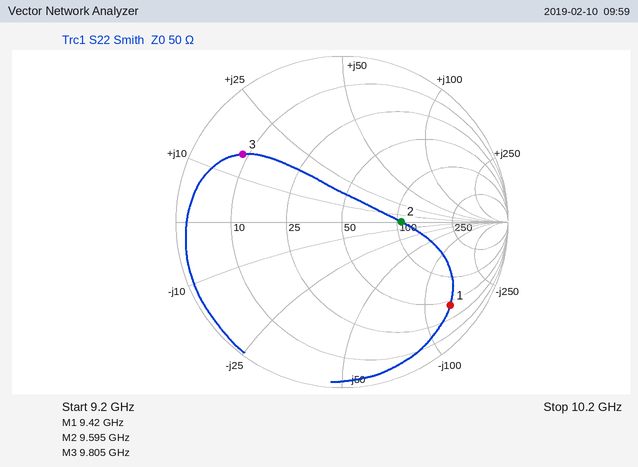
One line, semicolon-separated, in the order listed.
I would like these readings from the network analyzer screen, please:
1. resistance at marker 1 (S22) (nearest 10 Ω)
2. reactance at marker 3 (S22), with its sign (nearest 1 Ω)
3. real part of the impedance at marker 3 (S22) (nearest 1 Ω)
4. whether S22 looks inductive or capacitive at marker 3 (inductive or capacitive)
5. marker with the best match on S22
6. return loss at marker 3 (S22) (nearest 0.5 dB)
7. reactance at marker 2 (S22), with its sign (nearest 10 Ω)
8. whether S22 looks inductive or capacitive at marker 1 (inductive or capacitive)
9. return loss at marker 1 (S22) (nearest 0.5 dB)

40 Ω; +15 Ω; 9 Ω; inductive; marker 2; 3.0 dB; 0 Ω; capacitive; 1.5 dB
